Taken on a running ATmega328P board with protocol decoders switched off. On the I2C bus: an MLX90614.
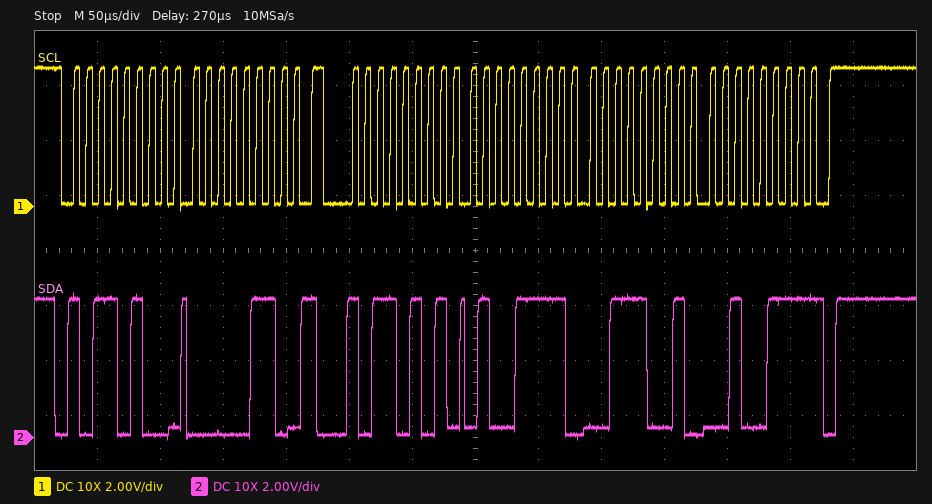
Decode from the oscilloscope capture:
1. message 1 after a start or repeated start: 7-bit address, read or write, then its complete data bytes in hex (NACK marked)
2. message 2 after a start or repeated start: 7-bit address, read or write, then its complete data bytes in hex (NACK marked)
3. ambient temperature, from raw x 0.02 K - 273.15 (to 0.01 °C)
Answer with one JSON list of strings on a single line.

["0x5A write: 06", "0x5A read: 4F 39 27 NACK", "20.27 °C"]
